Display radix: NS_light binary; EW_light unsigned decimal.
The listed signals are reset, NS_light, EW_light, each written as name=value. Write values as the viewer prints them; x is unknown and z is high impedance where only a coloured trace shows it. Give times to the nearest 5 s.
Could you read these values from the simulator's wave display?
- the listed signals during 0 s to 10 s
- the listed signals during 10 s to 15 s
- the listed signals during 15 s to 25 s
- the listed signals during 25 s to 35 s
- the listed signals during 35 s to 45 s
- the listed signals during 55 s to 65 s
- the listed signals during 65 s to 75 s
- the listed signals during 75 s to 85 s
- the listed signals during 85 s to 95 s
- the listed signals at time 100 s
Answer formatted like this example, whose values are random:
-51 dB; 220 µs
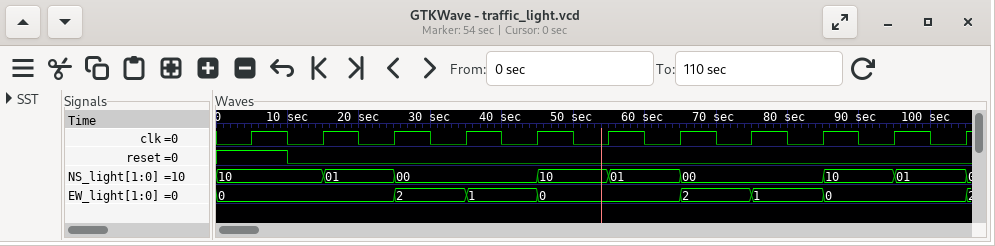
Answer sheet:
reset=1, NS_light=10, EW_light=0; reset=0, NS_light=10, EW_light=0; reset=0, NS_light=01, EW_light=0; reset=0, NS_light=00, EW_light=2; reset=0, NS_light=00, EW_light=1; reset=0, NS_light=01, EW_light=0; reset=0, NS_light=00, EW_light=2; reset=0, NS_light=00, EW_light=1; reset=0, NS_light=10, EW_light=0; reset=0, NS_light=01, EW_light=0
